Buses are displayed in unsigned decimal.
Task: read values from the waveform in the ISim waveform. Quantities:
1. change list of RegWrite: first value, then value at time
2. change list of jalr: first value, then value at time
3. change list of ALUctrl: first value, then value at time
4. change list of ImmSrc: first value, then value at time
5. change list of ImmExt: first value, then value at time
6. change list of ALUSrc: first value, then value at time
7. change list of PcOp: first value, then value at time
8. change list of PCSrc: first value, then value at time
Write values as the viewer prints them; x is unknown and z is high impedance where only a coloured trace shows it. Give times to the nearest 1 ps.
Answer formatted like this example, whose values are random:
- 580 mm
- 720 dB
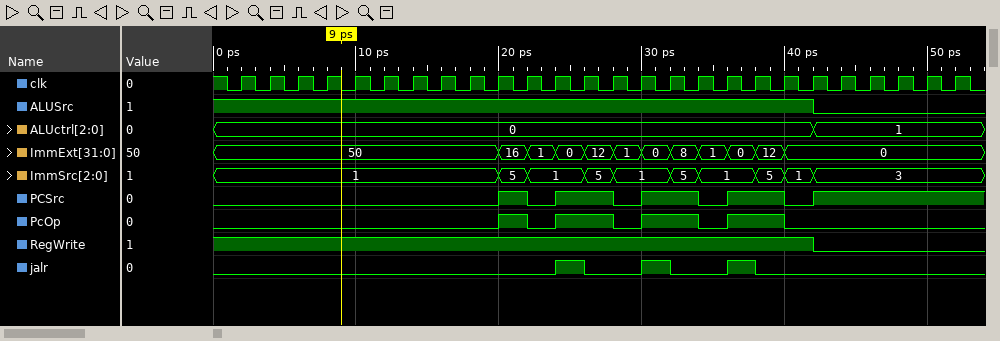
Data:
- 1, 0 at 42 ps
- 0, 1 at 24 ps, 0 at 26 ps, 1 at 30 ps, 0 at 32 ps, 1 at 36 ps, 0 at 38 ps
- 0, 1 at 42 ps
- 1, 5 at 20 ps, 1 at 22 ps, 5 at 26 ps, 1 at 28 ps, 5 at 32 ps, 1 at 34 ps, 5 at 38 ps, 1 at 40 ps, 3 at 42 ps
- 50, 16 at 20 ps, 1 at 22 ps, 0 at 24 ps, 12 at 26 ps, 1 at 28 ps, 0 at 30 ps, 8 at 32 ps, 1 at 34 ps, 0 at 36 ps, 12 at 38 ps, 0 at 40 ps
- 1, 0 at 42 ps
- 0, 1 at 20 ps, 0 at 22 ps, 1 at 24 ps, 0 at 28 ps, 1 at 30 ps, 0 at 34 ps, 1 at 36 ps, 0 at 40 ps
- 0, 1 at 20 ps, 0 at 22 ps, 1 at 24 ps, 0 at 28 ps, 1 at 30 ps, 0 at 34 ps, 1 at 36 ps, 0 at 40 ps, 1 at 42 ps
